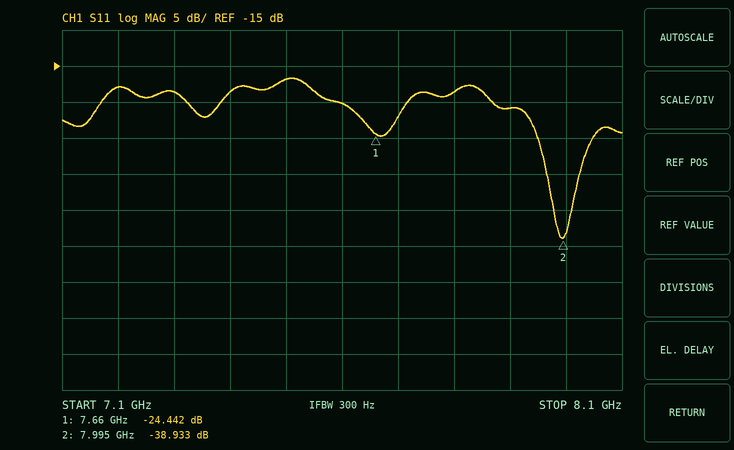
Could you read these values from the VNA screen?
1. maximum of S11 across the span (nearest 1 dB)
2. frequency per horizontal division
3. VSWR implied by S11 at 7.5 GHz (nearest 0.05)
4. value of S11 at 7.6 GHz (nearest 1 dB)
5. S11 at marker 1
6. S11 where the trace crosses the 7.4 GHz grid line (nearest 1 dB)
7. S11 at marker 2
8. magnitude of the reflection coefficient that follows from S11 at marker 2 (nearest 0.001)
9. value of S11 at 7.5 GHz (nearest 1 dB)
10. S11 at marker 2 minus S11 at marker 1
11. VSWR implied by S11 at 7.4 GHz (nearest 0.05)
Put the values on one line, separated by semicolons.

-17 dB; 100 MHz; 1.35; -20 dB; -24.442 dB; -19 dB; -38.933 dB; 0.011; -17 dB; -14.491 dB; 1.25
